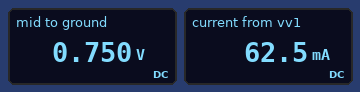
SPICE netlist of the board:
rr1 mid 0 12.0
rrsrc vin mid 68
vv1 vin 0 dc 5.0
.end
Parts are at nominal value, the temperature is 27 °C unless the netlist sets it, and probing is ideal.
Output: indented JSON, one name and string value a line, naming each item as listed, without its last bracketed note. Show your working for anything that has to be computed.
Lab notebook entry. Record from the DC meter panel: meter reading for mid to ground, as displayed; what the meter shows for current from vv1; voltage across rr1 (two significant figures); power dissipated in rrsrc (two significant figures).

{
  "meter reading for mid to ground, as displayed": "0.750 V",
  "what the meter shows for current from vv1": "62.5 mA",
  "voltage across rr1": "750 mV = 750 mV",
  "power dissipated in rrsrc": "(5 V - 750 mV)^2 / 68 Ω = 270 mW"
}
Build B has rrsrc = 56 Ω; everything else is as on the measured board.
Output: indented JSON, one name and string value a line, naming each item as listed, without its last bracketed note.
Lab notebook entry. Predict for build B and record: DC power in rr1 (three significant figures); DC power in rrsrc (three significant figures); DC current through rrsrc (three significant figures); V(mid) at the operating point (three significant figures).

{
  "DC power in rr1": "64.9 mW",
  "DC power in rrsrc": "303 mW",
  "DC current through rrsrc": "73.5 mA",
  "V(mid) at the operating point": "882 mV"
}
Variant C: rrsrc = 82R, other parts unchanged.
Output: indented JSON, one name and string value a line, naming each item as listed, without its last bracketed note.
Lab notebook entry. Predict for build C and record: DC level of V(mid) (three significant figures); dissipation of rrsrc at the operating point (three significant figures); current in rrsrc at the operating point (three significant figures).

{
  "DC level of V(mid)": "638 mV",
  "dissipation of rrsrc at the operating point": "232 mW",
  "current in rrsrc at the operating point": "53.2 mA"
}
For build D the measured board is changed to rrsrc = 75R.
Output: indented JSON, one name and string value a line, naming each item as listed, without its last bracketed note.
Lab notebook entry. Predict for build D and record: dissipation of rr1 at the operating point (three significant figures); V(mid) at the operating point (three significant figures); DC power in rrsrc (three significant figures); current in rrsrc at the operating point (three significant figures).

{
  "dissipation of rr1 at the operating point": "39.6 mW",
  "V(mid) at the operating point": "690 mV",
  "DC power in rrsrc": "248 mW",
  "current in rrsrc at the operating point": "57.5 mA"
}
